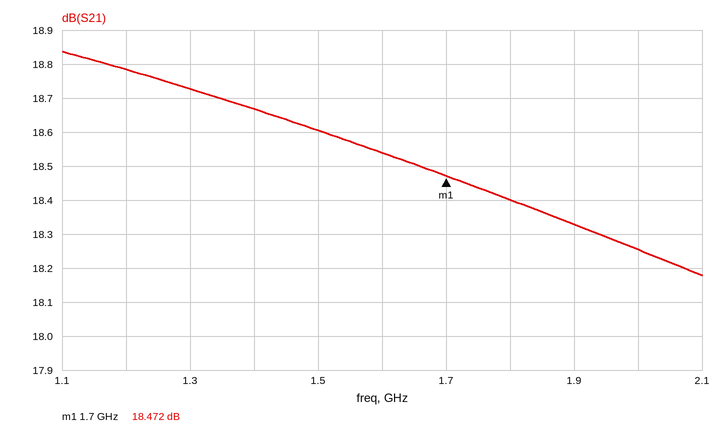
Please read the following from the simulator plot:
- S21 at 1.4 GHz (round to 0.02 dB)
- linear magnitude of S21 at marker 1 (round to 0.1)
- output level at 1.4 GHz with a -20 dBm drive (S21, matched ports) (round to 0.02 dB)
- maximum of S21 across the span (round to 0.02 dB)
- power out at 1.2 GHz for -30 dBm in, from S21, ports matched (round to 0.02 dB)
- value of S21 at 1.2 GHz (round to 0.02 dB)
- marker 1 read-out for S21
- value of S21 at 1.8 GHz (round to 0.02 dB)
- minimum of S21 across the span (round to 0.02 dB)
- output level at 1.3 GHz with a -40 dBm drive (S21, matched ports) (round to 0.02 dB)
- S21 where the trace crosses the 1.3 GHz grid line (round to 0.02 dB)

18.66 dB
8.4
-1.34 dBm
18.84 dB
-11.22 dBm
18.78 dB
18.472 dB
18.40 dB
18.18 dB
-21.28 dBm
18.72 dB
